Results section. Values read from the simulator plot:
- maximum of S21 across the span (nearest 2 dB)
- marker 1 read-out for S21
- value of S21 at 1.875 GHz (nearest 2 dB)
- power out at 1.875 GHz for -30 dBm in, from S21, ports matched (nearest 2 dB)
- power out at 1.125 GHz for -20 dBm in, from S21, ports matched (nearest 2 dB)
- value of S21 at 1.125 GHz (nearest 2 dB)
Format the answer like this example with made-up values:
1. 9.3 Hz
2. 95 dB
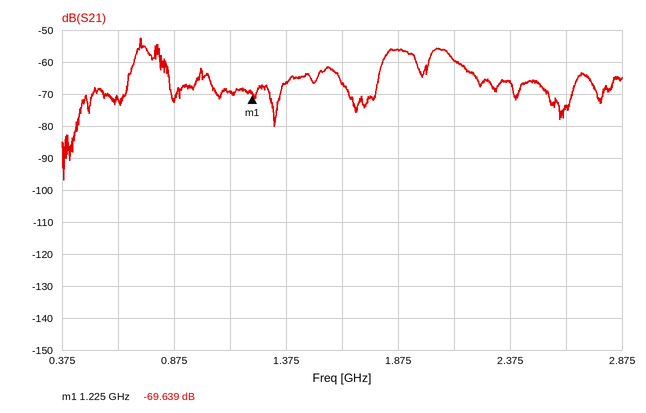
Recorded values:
1. -52 dB
2. -69.639 dB
3. -56 dB
4. -86 dBm
5. -90 dBm
6. -70 dB
